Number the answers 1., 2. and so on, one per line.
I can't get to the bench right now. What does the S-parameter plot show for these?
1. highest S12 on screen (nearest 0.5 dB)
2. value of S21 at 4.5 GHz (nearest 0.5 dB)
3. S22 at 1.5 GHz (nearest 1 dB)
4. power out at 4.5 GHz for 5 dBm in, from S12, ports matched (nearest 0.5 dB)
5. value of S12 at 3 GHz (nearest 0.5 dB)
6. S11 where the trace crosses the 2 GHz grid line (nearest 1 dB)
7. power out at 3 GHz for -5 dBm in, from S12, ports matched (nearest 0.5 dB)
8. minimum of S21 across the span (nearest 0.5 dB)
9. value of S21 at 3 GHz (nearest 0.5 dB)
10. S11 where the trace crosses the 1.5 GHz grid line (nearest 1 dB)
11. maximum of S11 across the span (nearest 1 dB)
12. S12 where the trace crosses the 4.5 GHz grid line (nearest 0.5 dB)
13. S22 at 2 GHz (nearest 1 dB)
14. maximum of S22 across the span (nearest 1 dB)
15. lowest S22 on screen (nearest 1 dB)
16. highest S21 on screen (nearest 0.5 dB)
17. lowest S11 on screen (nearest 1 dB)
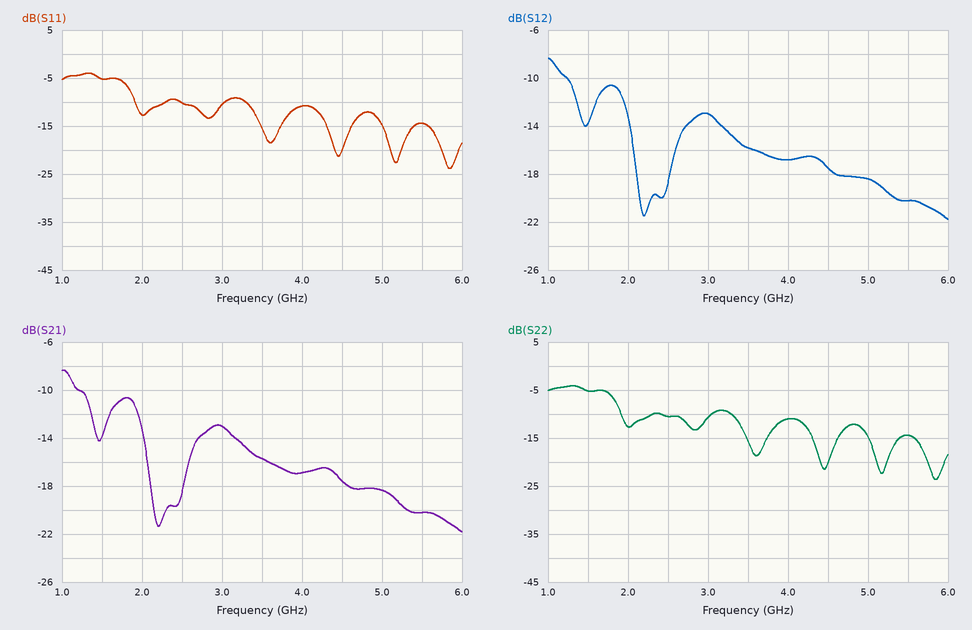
1. -8.5 dB
2. -17.5 dB
3. -5 dB
4. -12.5 dBm
5. -13.0 dB
6. -13 dB
7. -18.0 dBm
8. -22.0 dB
9. -13.0 dB
10. -5 dB
11. -4 dB
12. -17.5 dB
13. -13 dB
14. -4 dB
15. -24 dB
16. -8.5 dB
17. -24 dB
